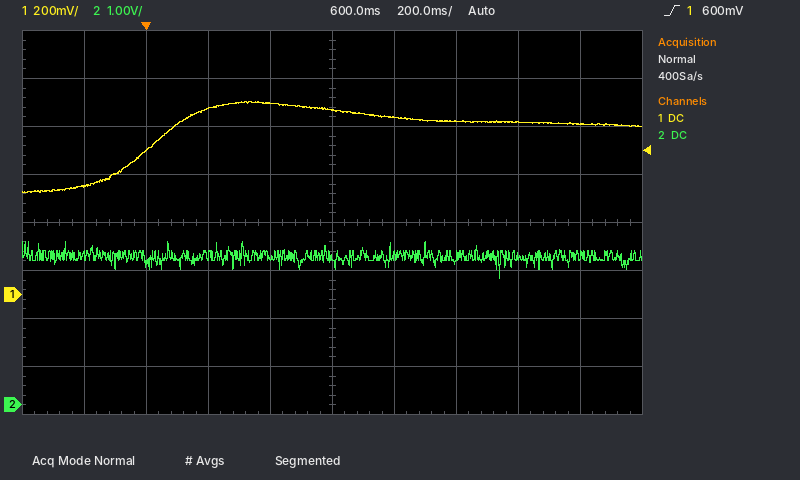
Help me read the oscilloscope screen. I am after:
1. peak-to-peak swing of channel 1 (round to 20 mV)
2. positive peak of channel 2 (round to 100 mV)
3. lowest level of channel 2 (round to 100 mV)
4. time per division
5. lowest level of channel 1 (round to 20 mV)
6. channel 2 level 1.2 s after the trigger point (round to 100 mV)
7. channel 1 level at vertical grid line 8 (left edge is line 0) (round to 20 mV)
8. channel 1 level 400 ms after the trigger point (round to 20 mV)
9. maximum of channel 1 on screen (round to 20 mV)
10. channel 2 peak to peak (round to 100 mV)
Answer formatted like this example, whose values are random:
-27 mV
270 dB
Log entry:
380 mV
3.4 V
2.6 V
200 ms
420 mV
3.1 V
720 mV
800 mV
800 mV
800 mV
